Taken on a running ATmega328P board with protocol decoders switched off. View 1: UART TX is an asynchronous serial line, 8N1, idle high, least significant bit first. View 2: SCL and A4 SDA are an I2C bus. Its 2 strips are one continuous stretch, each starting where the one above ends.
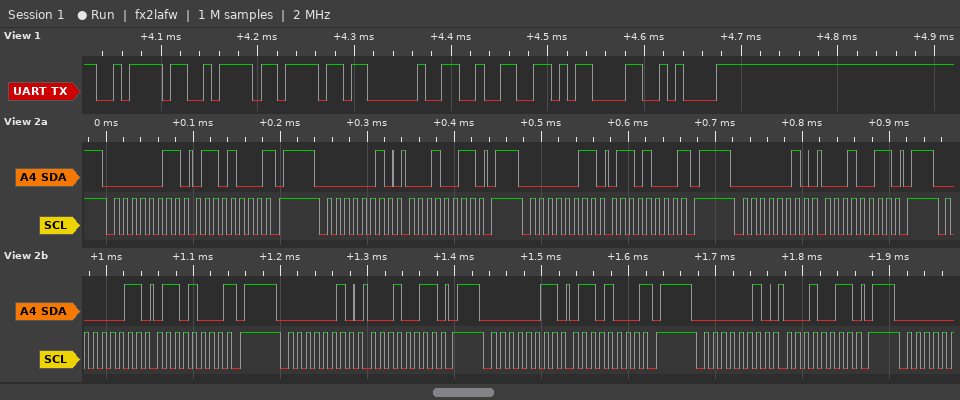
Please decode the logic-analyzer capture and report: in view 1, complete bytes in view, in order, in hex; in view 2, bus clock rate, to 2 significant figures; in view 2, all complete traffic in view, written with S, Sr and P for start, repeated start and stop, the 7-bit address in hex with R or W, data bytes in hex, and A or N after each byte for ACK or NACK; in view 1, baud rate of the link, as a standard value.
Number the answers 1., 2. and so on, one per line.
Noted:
1. 7A 7A 6F 20 32 0D 0A
2. 100 kHz
3. S 01R A 68 N P S 01W A 13 A P S 01R A 68 N P S 01W A 13 A P S 01R A 68 N P S 01W A 13 A P S 01R A 68 N P S 01W A 13 A P
4. 115200 baud
